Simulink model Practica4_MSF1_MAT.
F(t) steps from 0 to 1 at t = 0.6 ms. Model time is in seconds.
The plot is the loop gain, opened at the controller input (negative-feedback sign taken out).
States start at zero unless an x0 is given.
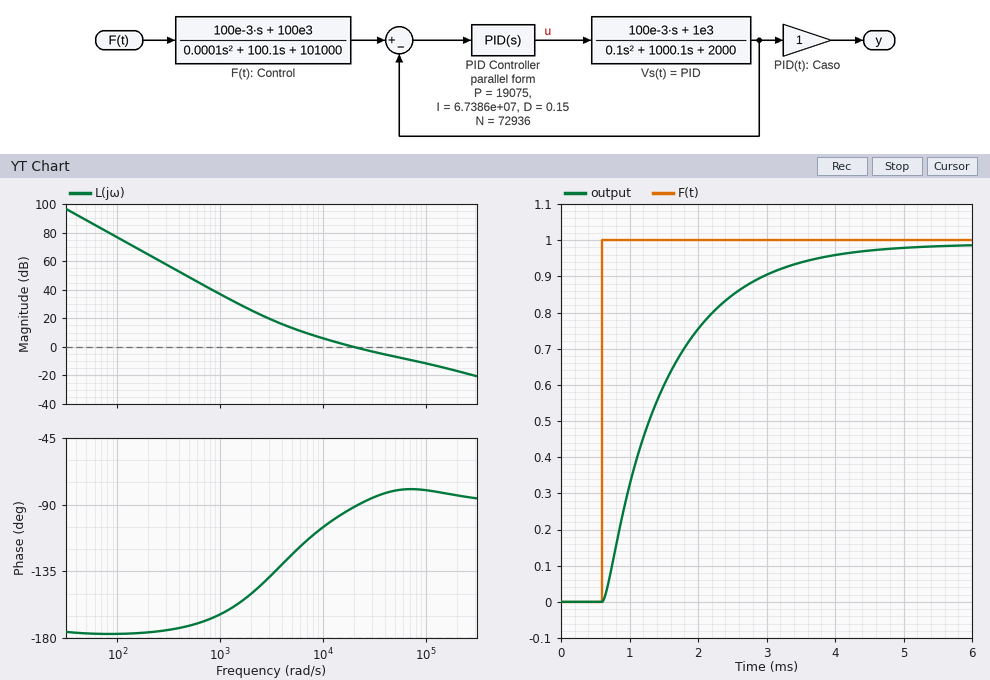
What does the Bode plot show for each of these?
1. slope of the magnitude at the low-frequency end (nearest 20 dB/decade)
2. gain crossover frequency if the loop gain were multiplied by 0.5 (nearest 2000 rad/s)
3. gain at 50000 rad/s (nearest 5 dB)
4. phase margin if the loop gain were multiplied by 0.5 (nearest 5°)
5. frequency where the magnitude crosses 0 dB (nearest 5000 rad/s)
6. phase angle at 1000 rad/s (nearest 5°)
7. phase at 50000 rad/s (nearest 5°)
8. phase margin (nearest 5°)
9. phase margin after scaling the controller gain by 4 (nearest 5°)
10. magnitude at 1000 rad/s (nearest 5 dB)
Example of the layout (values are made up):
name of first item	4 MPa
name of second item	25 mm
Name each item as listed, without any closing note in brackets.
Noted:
slope of the magnitude at the low-frequency end	-40 dB/decade
gain crossover frequency if the loop gain were multiplied by 0.5	10000 rad/s
gain at 50000 rad/s	-5 dB
phase margin if the loop gain were multiplied by 0.5	75°
frequency where the magnitude crosses 0 dB	20000 rad/s
phase angle at 1000 rad/s	-165°
phase at 50000 rad/s	-80°
phase margin	90°
phase margin after scaling the controller gain by 4	100°
magnitude at 1000 rad/s	35 dB
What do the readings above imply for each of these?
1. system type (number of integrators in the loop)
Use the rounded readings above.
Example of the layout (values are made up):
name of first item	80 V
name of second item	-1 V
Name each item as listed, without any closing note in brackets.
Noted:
system type	2
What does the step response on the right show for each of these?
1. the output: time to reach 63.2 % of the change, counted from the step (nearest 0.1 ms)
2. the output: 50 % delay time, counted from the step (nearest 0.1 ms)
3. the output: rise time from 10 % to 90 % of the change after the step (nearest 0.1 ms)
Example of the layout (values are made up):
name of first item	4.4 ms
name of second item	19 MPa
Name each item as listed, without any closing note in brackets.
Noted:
the output: time to reach 63.2 % of the change, counted from the step	1.0 ms
the output: 50 % delay time, counted from the step	0.7 ms
the output: rise time from 10 % to 90 % of the change after the step	2.1 ms
